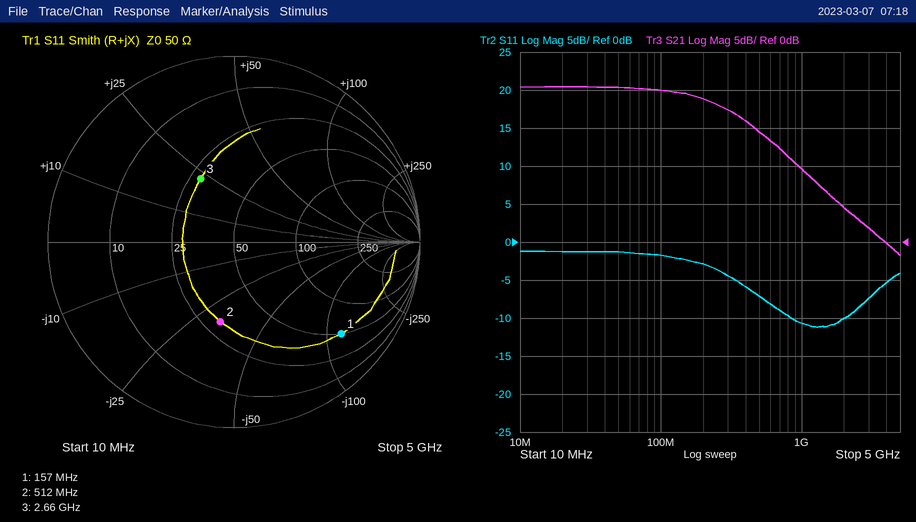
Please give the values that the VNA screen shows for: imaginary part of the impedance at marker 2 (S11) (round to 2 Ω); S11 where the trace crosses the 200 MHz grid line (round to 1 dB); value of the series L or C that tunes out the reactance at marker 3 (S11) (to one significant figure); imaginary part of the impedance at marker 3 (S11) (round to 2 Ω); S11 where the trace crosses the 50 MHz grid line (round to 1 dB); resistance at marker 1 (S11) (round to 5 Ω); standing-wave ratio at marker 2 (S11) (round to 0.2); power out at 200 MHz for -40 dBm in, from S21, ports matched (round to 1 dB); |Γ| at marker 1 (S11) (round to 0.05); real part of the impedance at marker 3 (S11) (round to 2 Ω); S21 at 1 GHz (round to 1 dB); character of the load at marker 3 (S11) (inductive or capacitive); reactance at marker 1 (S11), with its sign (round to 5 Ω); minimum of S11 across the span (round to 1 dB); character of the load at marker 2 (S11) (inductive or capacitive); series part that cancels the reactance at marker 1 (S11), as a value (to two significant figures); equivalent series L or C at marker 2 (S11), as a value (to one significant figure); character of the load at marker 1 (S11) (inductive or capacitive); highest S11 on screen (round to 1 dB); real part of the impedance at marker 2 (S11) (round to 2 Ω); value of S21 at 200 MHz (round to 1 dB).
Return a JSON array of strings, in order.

["-32 Ω", "-3 dB", "3 pF", "+22 Ω", "-1 dB", "50 Ω", "2.6", "-21 dBm", "0.75", "28 Ω", "10 dB", "inductive", "-115 Ω", "-11 dB", "capacitive", "120 nH", "10 pF", "capacitive", "-1 dB", "30 Ω", "19 dB"]
